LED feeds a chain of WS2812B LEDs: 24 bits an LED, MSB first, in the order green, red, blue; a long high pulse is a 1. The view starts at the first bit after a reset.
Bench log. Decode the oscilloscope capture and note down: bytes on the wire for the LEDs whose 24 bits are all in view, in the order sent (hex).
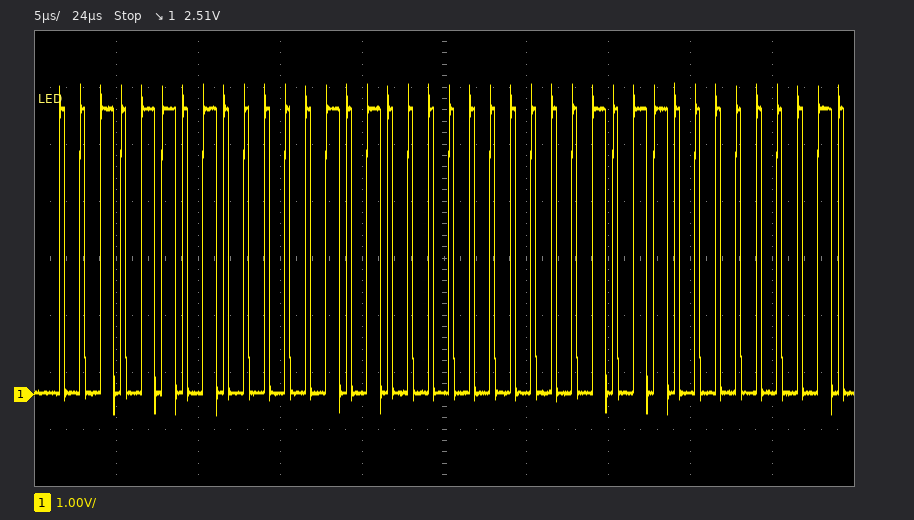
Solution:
2D 05 00
